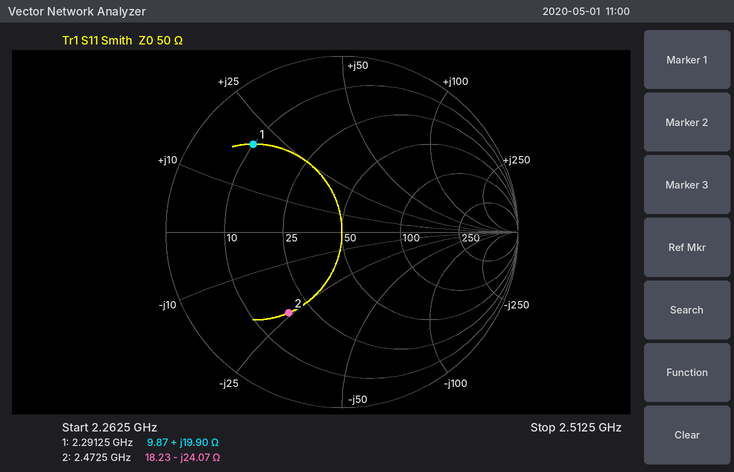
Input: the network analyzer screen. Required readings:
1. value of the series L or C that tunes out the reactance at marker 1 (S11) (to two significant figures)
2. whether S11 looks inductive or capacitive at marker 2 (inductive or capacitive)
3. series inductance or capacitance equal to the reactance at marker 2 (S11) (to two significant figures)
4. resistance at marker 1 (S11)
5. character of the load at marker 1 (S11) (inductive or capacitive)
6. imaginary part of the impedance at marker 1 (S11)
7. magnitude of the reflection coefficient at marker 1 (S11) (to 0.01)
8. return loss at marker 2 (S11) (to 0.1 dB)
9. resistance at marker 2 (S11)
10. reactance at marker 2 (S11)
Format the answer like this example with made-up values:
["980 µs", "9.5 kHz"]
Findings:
["3.5 pF", "capacitive", "2.7 pF", "9.87 Ω", "inductive", "+19.90 Ω", "0.71", "5.2 dB", "18.23 Ω", "-24.07 Ω"]
